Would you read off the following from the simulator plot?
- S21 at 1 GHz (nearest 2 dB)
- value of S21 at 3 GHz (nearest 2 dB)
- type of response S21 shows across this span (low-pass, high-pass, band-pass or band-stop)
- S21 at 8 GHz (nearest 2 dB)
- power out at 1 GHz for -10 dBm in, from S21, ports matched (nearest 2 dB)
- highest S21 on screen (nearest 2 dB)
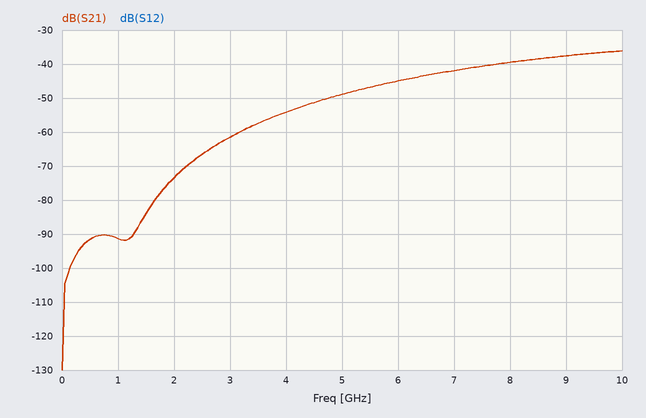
-92 dB
-62 dB
high-pass
-40 dB
-102 dBm
-36 dB
